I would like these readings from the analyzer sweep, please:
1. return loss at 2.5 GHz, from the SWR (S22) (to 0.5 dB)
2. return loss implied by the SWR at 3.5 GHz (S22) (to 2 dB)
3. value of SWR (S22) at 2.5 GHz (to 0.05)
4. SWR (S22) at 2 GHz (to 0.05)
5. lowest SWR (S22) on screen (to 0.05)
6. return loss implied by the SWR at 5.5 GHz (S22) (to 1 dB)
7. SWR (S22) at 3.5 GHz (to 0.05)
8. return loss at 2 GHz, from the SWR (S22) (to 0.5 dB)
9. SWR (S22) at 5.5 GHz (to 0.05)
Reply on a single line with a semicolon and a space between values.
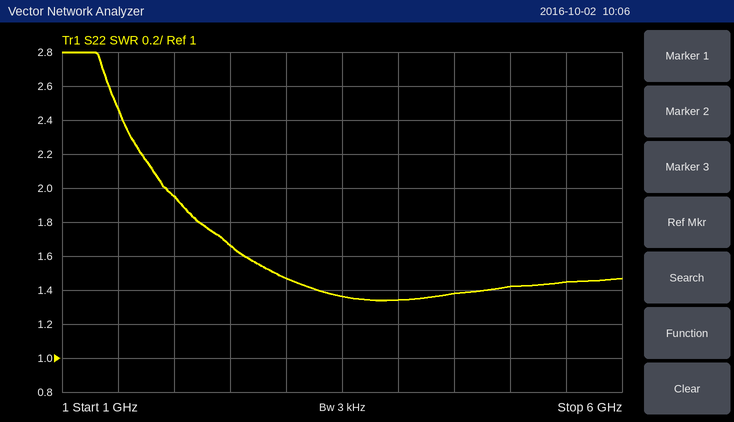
12.0 dB; 16 dB; 1.65; 1.95; 1.35; 15 dB; 1.35; 10.0 dB; 1.45
